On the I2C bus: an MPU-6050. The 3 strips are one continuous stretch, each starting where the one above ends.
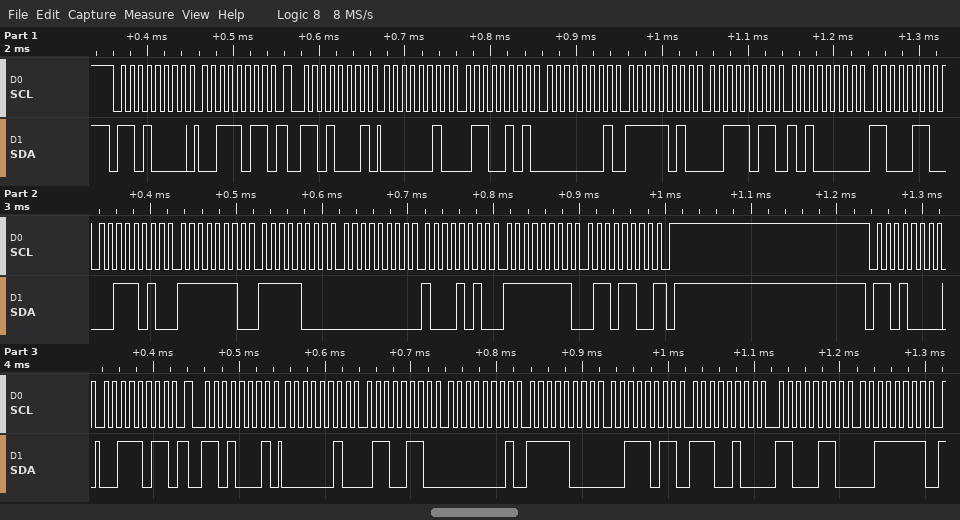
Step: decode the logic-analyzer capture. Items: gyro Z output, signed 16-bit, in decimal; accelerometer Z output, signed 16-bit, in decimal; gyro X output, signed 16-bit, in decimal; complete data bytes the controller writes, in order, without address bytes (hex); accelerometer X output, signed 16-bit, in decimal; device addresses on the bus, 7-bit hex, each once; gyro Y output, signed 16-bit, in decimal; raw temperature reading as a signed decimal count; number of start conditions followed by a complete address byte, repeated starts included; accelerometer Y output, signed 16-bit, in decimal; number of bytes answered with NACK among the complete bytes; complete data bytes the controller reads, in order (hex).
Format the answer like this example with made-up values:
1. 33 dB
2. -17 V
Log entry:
1. -148
2. 15264
3. -264
4. 3B 3B
5. 613
6. 0x68
7. 138
8. -14790
9. 4
10. 506
11. 1
12. 02 65 01 FA 3B A0 C6 3A FE F8 00 8A FF 6C 02 66 01 F8 3B E4 C6 3F
